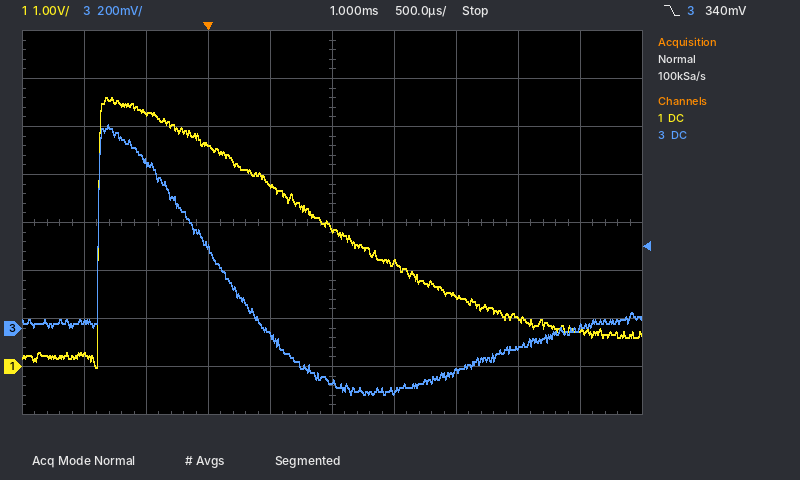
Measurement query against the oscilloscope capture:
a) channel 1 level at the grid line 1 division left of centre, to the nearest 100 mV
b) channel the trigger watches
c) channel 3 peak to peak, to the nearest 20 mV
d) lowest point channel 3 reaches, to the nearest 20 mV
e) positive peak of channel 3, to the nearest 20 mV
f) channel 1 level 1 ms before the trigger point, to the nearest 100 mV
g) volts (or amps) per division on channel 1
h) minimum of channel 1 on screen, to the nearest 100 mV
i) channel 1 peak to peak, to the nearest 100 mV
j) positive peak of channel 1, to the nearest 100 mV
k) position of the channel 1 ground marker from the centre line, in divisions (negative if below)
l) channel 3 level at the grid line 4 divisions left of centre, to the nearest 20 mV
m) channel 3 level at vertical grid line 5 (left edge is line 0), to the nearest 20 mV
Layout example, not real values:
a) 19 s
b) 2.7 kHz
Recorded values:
a) 3.8 V
b) channel 3
c) 1.12 V
d) -280 mV
e) 840 mV
f) 300 mV
g) 1 V
h) 0.0 V
i) 5.6 V
j) 5.6 V
k) -3.0 div
l) 20 mV
m) -220 mV
